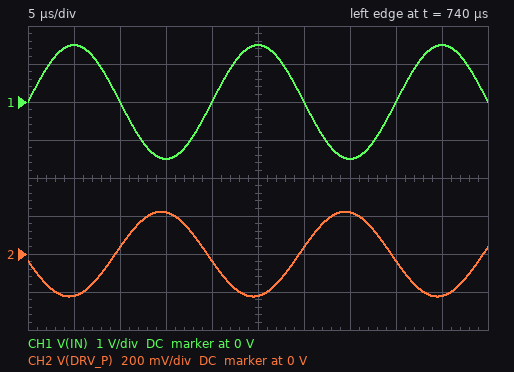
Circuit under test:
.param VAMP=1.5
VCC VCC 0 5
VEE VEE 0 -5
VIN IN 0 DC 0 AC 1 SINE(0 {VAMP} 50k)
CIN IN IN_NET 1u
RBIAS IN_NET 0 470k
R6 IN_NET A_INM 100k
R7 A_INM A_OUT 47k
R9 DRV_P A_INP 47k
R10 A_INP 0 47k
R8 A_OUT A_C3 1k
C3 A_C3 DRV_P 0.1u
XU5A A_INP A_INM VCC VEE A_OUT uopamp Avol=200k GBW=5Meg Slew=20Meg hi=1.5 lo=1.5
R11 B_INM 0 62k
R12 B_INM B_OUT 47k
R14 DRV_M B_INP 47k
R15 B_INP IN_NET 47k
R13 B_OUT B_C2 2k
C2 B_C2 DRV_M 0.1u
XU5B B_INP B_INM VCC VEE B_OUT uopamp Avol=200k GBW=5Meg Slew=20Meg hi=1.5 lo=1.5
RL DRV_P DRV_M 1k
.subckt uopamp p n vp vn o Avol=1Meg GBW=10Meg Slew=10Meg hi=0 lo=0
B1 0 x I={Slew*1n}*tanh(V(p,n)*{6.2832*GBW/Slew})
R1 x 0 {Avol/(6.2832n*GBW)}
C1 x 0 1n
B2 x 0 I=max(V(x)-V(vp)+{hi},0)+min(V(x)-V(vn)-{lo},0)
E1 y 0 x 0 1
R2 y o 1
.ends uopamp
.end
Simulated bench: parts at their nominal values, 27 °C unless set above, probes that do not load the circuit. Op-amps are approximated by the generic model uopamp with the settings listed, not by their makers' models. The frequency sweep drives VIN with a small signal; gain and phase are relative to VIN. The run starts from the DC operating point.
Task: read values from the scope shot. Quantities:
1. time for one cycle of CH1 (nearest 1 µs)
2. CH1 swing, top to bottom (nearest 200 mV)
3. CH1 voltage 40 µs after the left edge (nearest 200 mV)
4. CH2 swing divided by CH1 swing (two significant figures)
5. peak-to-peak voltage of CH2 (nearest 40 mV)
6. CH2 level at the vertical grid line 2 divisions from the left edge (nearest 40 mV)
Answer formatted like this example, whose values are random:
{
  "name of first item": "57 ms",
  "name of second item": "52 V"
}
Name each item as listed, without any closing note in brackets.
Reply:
{
  "time for one cycle of CH1": "20 µs",
  "CH1 swing, top to bottom": "3.0 V",
  "CH1 voltage 40 µs after the left edge": "0 V",
  "CH2 swing divided by CH1 swing": "0.15",
  "peak-to-peak voltage of CH2": "440 mV",
  "CH2 level at the vertical grid line 2 divisions from the left edge": "40 mV"
}
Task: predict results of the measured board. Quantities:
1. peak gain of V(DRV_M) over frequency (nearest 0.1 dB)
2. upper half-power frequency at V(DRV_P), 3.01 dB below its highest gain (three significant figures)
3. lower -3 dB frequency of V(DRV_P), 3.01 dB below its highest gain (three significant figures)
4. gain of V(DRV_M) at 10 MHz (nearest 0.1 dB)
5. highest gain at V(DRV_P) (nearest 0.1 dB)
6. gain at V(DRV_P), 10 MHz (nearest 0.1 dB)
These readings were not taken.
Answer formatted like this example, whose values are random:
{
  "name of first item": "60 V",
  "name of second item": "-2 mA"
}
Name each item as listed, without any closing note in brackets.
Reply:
{
  "peak gain of V(DRV_M) over frequency": "0 dB",
  "upper half-power frequency at V(DRV_P), 3.01 dB below its highest gain": "1.06 kHz",
  "lower -3 dB frequency of V(DRV_P), 3.01 dB below its highest gain": "47.9 Hz",
  "gain of V(DRV_M) at 10 MHz": "-26.2 dB",
  "highest gain at V(DRV_P)": "-0.2 dB",
  "gain at V(DRV_P), 10 MHz": "-25.6 dB"
}
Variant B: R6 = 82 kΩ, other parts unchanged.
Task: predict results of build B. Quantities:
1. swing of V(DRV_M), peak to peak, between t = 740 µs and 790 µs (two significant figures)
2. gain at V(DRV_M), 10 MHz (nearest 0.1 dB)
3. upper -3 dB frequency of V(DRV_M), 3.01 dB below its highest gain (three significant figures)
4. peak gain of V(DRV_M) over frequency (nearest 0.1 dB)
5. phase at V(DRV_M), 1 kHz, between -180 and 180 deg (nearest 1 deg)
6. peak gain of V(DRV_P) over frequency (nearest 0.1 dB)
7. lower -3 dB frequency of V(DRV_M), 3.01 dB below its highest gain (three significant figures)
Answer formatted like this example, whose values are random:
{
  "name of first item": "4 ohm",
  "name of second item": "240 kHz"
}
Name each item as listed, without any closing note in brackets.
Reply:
{
  "swing of V(DRV_M), peak to peak, between t = 740 µs and 790 µs": "210 mV",
  "gain at V(DRV_M), 10 MHz": "-28.1 dB",
  "upper -3 dB frequency of V(DRV_M), 3.01 dB below its highest gain": "1.09 kHz",
  "peak gain of V(DRV_M) over frequency": "-1.1 dB",
  "phase at V(DRV_M), 1 kHz, between -180 and 180 deg": "-49 deg",
  "peak gain of V(DRV_P) over frequency": "-1.2 dB",
  "lower -3 dB frequency of V(DRV_M), 3.01 dB below its highest gain": "46.7 Hz"
}
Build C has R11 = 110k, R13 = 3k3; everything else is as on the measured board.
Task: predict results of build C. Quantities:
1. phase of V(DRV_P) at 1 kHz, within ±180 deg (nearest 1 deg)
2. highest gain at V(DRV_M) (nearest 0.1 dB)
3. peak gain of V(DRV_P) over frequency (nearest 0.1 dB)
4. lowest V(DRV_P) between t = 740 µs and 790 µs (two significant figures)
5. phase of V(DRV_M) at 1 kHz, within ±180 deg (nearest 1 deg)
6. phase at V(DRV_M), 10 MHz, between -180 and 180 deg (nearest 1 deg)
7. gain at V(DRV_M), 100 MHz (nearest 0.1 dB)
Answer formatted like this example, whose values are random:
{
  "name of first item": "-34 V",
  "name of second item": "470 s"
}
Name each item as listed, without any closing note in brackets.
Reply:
{
  "phase of V(DRV_P) at 1 kHz, within ±180 deg": "-116 deg",
  "highest gain at V(DRV_M)": "-5.6 dB",
  "peak gain of V(DRV_P) over frequency": "-2.8 dB",
  "lowest V(DRV_P) between t = 740 µs and 790 µs": "-1.1 V",
  "phase of V(DRV_M) at 1 kHz, within ±180 deg": "-103 deg",
  "phase at V(DRV_M), 10 MHz, between -180 and 180 deg": "16 deg",
  "gain at V(DRV_M), 100 MHz": "-37.6 dB"
}
